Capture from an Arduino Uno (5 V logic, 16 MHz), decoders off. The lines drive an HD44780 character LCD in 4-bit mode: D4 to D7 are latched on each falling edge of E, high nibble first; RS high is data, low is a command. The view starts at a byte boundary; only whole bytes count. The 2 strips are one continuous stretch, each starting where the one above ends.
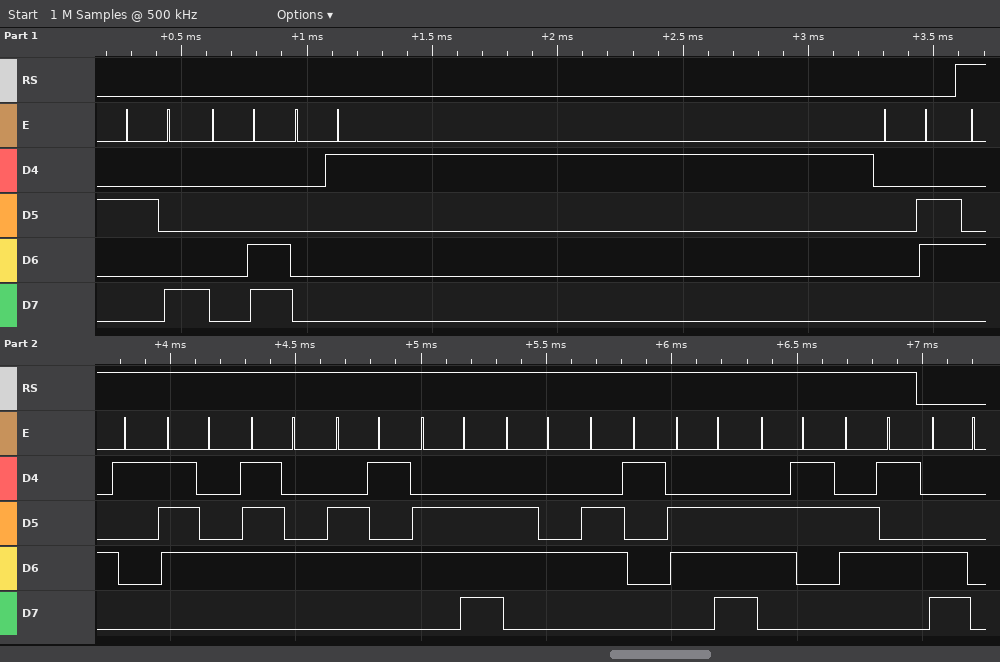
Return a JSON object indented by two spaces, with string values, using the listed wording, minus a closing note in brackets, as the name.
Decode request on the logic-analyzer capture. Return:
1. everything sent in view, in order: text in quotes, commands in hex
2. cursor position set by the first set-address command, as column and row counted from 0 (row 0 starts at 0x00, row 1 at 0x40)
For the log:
{
  "everything sent in view, in order: text in quotes, commands in hex": "0x28 0x0C 0x01 0x06 \"Attendance\" 0xC0",
  "cursor position set by the first set-address command, as column and row counted from 0": "column 0, row 1"
}
